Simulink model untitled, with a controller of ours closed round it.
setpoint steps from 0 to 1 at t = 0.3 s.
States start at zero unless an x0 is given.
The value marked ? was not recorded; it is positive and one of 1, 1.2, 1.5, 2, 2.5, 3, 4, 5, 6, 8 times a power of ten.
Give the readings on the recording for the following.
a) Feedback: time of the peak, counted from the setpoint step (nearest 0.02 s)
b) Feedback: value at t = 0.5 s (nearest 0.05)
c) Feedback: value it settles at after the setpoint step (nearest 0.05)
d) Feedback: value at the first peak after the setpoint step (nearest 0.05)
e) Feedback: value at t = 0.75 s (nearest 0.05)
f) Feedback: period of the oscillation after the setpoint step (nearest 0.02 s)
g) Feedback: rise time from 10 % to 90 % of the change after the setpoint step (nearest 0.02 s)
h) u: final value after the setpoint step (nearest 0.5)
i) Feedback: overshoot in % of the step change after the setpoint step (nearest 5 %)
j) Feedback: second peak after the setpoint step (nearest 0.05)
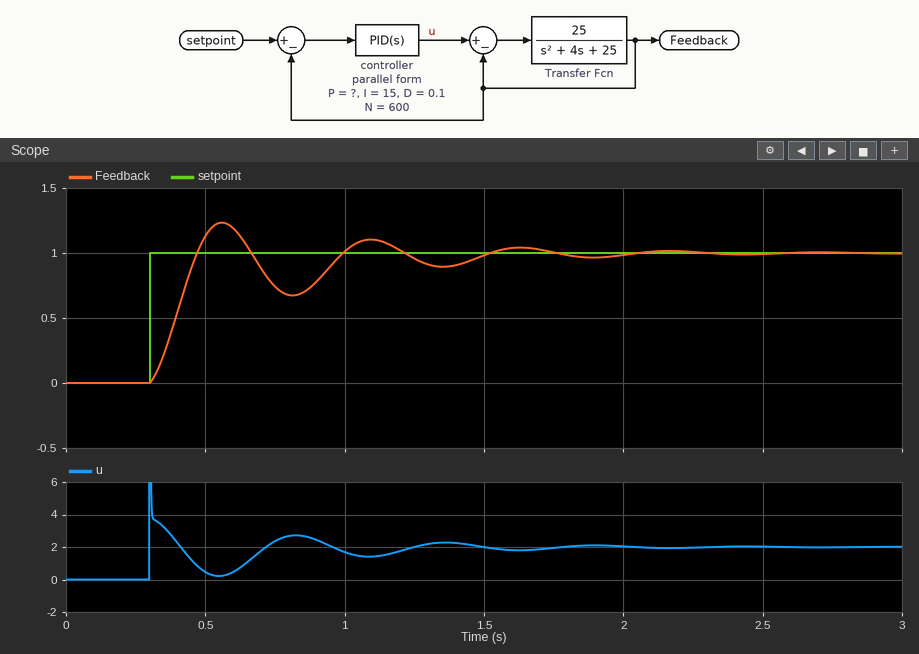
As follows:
0.26 s
1.15
1.00
1.25
0.75
0.54 s
0.12 s
2.0
25 %
1.10
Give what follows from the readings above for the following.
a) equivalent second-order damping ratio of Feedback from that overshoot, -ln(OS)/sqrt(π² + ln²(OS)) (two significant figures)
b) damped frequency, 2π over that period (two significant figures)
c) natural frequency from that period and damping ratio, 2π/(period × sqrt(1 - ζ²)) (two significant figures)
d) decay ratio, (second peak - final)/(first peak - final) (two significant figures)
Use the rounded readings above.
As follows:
0.40
12 rad/s
13 rad/s
0.40
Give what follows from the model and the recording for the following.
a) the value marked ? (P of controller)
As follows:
4
